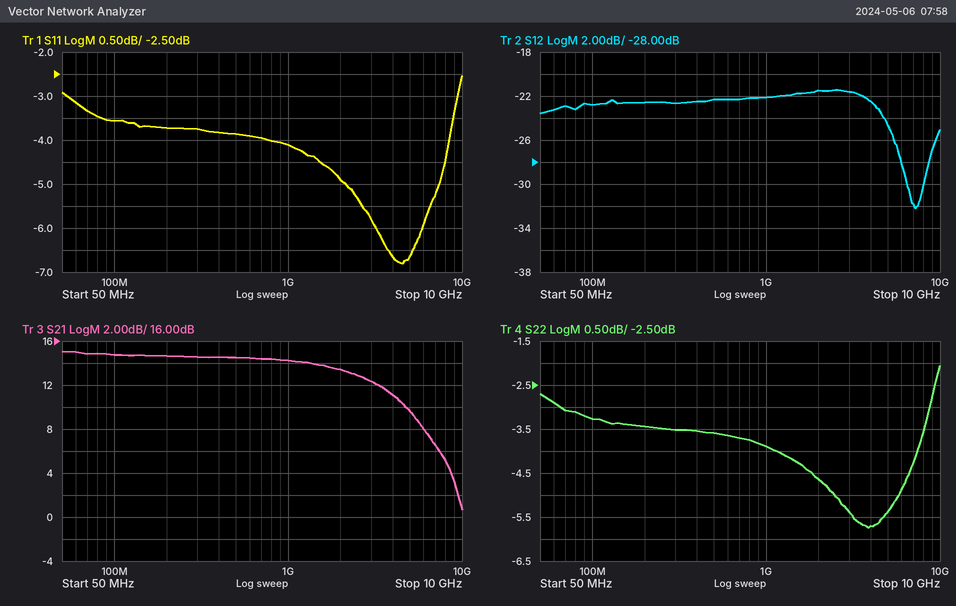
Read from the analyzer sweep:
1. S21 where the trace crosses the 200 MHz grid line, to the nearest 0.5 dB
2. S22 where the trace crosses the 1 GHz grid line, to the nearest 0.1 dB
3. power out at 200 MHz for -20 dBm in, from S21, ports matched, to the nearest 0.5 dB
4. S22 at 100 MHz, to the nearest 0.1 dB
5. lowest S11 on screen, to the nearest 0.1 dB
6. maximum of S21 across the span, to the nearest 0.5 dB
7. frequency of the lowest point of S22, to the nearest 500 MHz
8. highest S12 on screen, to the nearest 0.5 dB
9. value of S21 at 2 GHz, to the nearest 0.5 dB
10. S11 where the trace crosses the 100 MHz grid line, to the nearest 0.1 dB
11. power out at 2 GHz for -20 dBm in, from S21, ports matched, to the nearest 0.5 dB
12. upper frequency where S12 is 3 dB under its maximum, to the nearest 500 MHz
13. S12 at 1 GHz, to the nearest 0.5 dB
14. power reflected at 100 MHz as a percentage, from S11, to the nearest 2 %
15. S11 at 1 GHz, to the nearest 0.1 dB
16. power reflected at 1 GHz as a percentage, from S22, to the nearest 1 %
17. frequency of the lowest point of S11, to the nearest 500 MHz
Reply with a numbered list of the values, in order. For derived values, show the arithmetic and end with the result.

1. 14.5 dB
2. -3.9 dB
3. -20 dBm + (14.5 dB) = -5.5 dBm
4. -3.3 dB
5. -6.8 dB
6. 15.0 dB
7. 4.0 GHz
8. -21.5 dB
9. 13.5 dB
10. -3.6 dB
11. -20 dBm + (13.5 dB) = -6.5 dBm
12. 5.0 GHz
13. -22.0 dB
14. 10^(-3.6/10) ≈ 44 %
15. -4.1 dB
16. 10^(-3.9/10) ≈ 41 %
17. 4.5 GHz
